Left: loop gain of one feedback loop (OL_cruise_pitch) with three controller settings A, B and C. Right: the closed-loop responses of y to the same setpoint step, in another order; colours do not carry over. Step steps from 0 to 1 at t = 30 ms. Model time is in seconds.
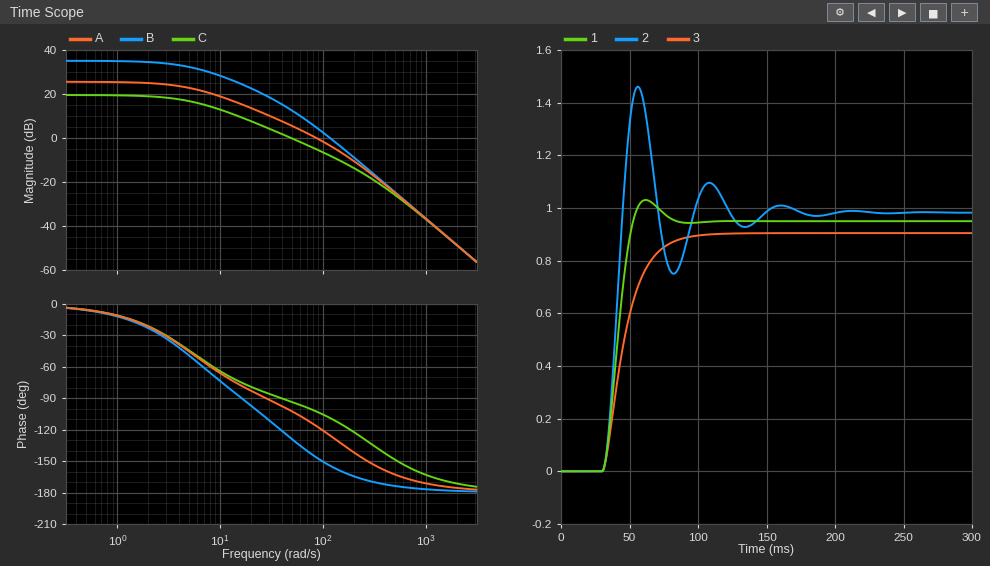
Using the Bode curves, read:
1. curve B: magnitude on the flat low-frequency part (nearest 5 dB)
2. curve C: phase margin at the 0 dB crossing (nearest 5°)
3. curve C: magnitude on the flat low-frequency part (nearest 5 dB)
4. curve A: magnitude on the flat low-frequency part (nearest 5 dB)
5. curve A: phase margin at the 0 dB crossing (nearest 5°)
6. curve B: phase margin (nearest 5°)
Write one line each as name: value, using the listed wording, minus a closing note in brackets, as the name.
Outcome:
curve B: magnitude on the flat low-frequency part: 35 dB
curve C: phase margin at the 0 dB crossing: 85°
curve C: magnitude on the flat low-frequency part: 20 dB
curve A: magnitude on the flat low-frequency part: 25 dB
curve A: phase margin at the 0 dB crossing: 65°
curve B: phase margin: 25°
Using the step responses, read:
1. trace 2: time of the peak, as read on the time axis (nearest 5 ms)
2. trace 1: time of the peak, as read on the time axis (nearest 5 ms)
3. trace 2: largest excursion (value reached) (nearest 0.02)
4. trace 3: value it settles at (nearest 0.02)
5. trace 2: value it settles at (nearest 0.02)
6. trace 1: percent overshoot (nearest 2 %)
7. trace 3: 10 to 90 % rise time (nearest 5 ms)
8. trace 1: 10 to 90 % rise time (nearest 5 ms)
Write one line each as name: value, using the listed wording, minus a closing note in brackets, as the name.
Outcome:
trace 2: time of the peak, as read on the time axis: 55 ms
trace 1: time of the peak, as read on the time axis: 60 ms
trace 2: largest excursion (value reached): 1.46
trace 3: value it settles at: 0.90
trace 2: value it settles at: 0.98
trace 1: percent overshoot: 8 %
trace 3: 10 to 90 % rise time: 35 ms
trace 1: 10 to 90 % rise time: 15 ms
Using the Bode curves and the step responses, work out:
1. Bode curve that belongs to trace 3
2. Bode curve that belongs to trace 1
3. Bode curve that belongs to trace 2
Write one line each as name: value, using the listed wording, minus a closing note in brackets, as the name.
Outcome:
Bode curve that belongs to trace 3: C
Bode curve that belongs to trace 1: A
Bode curve that belongs to trace 2: B
